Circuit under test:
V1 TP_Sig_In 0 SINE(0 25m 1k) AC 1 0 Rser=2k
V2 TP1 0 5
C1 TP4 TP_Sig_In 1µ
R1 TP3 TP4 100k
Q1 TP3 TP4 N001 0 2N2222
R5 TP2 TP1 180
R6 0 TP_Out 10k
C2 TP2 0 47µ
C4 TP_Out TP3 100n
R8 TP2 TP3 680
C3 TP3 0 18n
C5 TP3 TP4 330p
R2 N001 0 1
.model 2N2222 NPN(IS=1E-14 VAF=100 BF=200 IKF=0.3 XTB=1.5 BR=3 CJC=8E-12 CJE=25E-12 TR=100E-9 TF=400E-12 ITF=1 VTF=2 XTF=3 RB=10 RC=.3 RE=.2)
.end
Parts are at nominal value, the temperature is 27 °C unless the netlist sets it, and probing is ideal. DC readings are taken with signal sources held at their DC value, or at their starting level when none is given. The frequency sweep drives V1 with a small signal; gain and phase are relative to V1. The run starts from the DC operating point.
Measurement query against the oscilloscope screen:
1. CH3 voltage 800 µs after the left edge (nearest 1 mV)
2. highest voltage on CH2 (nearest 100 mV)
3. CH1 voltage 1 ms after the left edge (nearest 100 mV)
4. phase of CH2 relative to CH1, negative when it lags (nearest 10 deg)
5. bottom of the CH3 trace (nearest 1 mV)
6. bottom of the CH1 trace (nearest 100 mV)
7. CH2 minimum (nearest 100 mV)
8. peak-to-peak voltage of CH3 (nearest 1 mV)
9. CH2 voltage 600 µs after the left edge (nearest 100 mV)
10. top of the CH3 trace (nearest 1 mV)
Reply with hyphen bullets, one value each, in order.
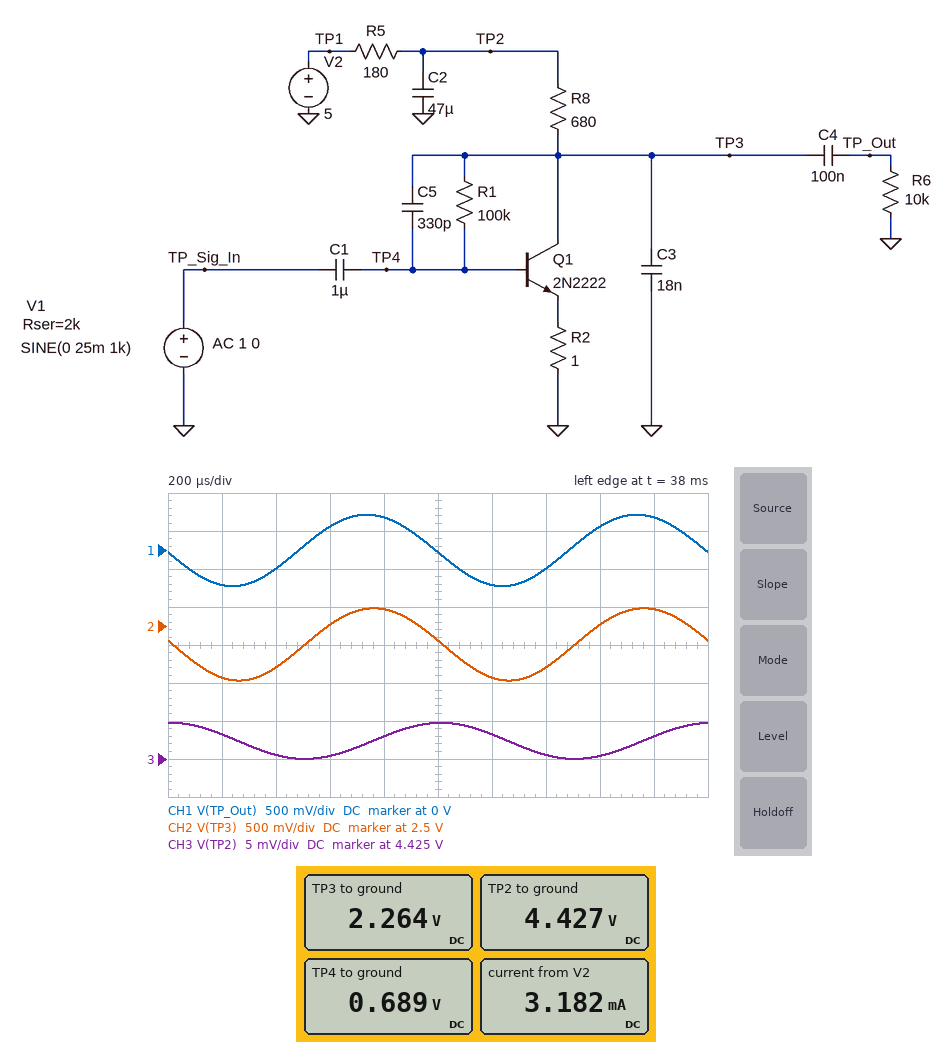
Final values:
- 4.428 V
- 2.7 V
- 0 V
- -10 deg
- 4.425 V
- -500 mV
- 1.8 V
- 5 mV
- 2.5 V
- 4.430 V
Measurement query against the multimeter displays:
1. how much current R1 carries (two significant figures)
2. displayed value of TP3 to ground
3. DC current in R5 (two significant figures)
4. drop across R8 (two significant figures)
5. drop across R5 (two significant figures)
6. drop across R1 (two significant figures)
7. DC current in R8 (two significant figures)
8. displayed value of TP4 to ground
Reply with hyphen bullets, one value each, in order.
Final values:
- 16 µA
- 2.264 V
- 3.2 mA
- 2.2 V
- 570 mV
- 1.6 V
- 3.2 mA
- 0.689 V
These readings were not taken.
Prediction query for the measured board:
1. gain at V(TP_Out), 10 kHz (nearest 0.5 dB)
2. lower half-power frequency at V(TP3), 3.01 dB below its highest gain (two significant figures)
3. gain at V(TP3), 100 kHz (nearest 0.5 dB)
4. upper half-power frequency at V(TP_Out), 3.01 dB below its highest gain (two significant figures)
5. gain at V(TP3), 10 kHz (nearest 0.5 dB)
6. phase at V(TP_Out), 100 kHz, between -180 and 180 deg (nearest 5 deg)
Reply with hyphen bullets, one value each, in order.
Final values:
- 21.5 dB
- 50 Hz
- 3.5 dB
- 8.3 kHz
- 21.5 dB
- 90 deg
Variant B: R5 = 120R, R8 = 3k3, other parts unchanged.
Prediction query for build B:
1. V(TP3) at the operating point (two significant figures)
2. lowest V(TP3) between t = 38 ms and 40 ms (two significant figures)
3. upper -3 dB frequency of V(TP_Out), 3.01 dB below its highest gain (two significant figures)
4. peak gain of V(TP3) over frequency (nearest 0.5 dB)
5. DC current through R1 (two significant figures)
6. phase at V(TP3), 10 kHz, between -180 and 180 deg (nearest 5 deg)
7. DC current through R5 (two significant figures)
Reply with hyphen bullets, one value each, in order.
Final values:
- 1.2 V
- 510 mV
- 4.5 kHz
- 29.0 dB
- 5.5 µA
- 110 deg
- 1.1 mA
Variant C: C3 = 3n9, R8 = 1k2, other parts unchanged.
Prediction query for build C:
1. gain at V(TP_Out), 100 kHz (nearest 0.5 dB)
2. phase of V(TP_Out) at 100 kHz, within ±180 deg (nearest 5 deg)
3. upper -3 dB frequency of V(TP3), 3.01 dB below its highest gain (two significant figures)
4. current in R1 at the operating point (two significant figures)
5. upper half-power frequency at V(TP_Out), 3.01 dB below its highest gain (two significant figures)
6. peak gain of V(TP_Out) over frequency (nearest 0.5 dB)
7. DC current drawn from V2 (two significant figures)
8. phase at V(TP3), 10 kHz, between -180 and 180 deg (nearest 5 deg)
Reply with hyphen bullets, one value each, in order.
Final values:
- 6.0 dB
- 95 deg
- 8.7 kHz
- 11 µA
- 9.0 kHz
- 27.5 dB
- 2.3 mA
- 130 deg
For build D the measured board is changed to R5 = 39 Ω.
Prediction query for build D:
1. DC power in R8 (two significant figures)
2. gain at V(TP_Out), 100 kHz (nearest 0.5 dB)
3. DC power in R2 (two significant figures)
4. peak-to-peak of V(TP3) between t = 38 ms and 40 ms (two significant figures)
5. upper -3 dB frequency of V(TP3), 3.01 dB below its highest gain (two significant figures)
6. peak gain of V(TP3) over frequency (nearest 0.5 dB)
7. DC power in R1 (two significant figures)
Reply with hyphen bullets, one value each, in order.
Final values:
- 8.6 mW
- 4.0 dB
- 13 µW
- 980 mV
- 7.9 kHz
- 26.0 dB
- 31 µW
